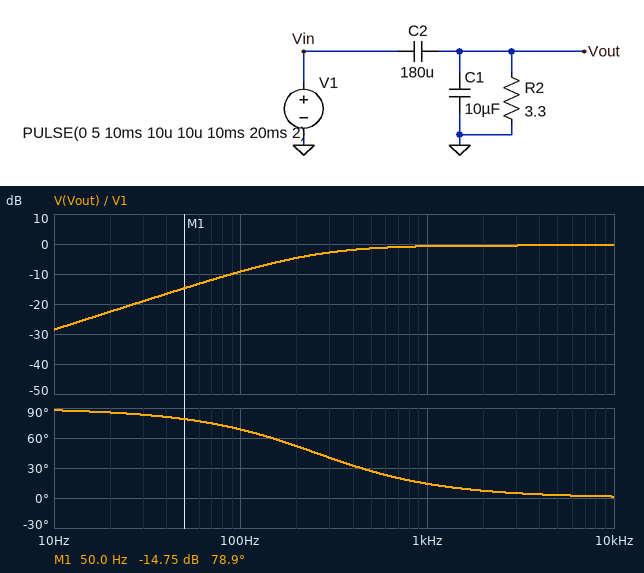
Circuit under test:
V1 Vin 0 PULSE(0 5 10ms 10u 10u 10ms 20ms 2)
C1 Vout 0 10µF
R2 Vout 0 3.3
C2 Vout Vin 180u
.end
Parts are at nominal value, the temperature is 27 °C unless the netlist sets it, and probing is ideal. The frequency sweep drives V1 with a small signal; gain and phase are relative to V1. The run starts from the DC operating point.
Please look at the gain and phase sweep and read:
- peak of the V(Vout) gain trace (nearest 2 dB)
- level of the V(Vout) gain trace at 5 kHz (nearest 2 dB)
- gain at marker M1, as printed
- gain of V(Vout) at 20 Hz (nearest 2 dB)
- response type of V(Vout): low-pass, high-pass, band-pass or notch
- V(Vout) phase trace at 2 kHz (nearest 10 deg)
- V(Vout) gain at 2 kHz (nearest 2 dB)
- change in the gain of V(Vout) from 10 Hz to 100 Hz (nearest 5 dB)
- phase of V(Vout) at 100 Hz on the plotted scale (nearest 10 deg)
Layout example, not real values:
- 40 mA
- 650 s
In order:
- 0 dB
- 0 dB
- -14.75 dB
- -22 dB
- high-pass
- 10 deg
- 0 dB
- 20 dB
- 70 deg
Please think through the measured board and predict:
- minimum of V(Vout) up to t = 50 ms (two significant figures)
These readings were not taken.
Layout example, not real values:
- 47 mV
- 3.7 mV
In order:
- -4.7 V
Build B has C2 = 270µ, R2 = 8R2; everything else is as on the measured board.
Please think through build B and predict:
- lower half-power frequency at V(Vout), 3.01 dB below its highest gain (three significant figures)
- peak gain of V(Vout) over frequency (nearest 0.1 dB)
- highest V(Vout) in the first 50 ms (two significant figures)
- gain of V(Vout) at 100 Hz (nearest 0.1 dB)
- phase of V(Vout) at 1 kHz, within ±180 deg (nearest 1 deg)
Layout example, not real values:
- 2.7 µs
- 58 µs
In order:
- 69.3 Hz
- -0.3 dB
- 4.8 V
- -2.0 dB
- 4 deg
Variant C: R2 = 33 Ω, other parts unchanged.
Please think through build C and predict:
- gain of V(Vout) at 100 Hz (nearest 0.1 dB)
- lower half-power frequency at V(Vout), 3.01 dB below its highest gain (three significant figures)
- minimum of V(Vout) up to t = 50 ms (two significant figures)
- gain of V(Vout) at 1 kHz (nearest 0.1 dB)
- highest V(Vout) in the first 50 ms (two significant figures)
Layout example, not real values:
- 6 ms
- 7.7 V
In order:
- -0.7 dB
- 25.4 Hz
- -3.9 V
- -0.5 dB
- 4.7 V
